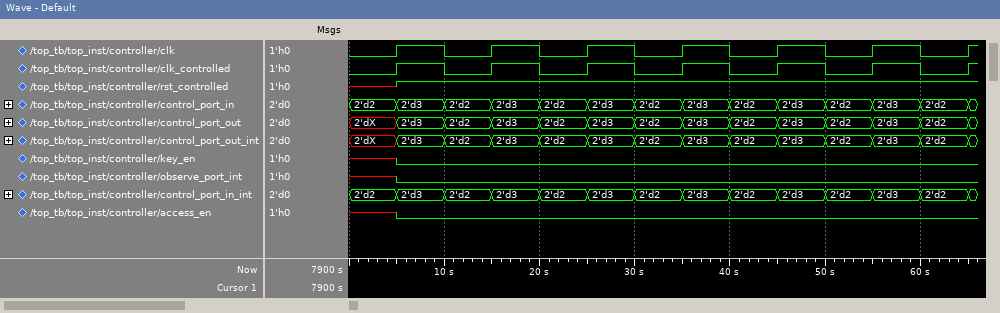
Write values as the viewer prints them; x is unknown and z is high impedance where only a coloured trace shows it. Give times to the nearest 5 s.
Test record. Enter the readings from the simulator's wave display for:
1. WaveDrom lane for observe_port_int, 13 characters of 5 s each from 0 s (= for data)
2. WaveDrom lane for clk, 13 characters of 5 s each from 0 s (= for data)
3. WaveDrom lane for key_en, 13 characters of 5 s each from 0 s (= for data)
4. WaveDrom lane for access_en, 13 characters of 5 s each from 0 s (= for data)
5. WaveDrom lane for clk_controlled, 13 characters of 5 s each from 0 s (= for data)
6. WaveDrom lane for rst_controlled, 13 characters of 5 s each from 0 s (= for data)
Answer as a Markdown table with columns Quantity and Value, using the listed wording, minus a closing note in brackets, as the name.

| Quantity | Value |
|---|---|
| WaveDrom lane for observe_port_int, 13 characters of 5 s each from 0 s | {name: 'observe_port_int', wave: 'x0...........'} |
| WaveDrom lane for clk, 13 characters of 5 s each from 0 s | {name: 'clk', wave: '0101010101010'} |
| WaveDrom lane for key_en, 13 characters of 5 s each from 0 s | {name: 'key_en', wave: 'x0...........'} |
| WaveDrom lane for access_en, 13 characters of 5 s each from 0 s | {name: 'access_en', wave: 'x0...........'} |
| WaveDrom lane for clk_controlled, 13 characters of 5 s each from 0 s | {name: 'clk_controlled', wave: '0101010101010'} |
| WaveDrom lane for rst_controlled, 13 characters of 5 s each from 0 s | {name: 'rst_controlled', wave: 'x1...........'} |
